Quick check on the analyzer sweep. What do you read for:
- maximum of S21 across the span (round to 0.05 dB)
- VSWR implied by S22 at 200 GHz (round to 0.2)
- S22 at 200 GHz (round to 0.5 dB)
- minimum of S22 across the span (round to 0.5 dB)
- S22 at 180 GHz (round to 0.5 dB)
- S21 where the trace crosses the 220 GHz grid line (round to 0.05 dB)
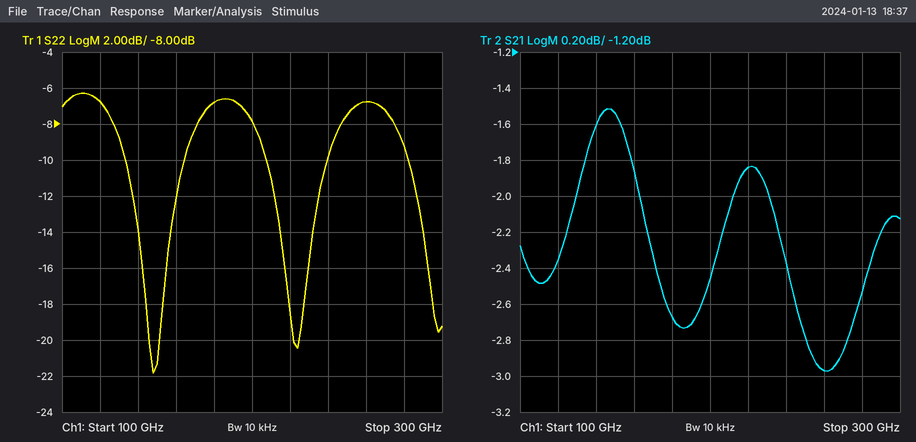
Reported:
-1.50 dB
2.4
-8.0 dB
-22.0 dB
-7.0 dB
-1.85 dB
